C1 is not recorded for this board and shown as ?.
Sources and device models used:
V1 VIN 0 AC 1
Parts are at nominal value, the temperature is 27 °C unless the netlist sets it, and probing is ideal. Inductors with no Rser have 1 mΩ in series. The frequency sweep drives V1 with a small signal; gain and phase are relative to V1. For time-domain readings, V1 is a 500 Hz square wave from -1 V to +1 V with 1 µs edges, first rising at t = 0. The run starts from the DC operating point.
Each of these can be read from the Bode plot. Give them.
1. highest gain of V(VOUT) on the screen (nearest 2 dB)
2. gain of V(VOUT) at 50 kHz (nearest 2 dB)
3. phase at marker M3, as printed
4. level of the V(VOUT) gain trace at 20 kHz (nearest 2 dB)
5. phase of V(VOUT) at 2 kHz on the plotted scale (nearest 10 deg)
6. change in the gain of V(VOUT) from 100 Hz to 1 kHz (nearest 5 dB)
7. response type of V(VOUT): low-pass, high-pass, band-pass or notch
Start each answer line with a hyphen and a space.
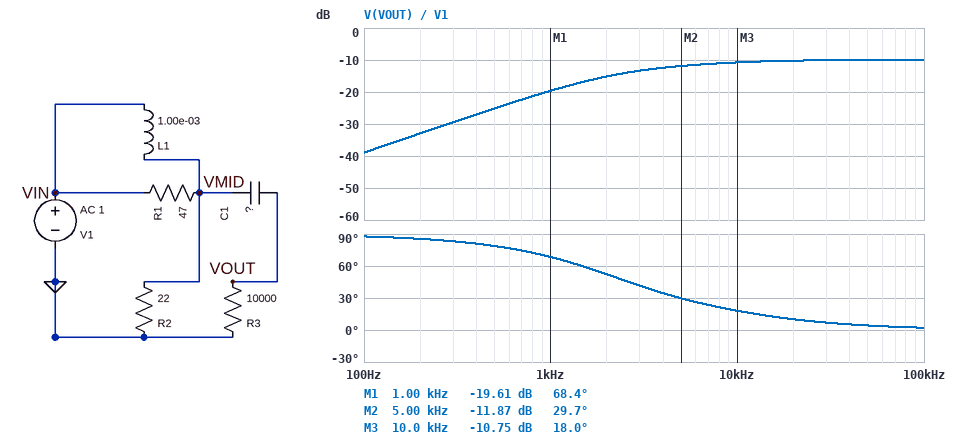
- -10 dB
- -10 dB
- 18.0 deg
- -10 dB
- 50 deg
- 20 dB
- high-pass
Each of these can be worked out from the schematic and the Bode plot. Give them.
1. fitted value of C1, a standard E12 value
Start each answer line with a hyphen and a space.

- 1.8 nF
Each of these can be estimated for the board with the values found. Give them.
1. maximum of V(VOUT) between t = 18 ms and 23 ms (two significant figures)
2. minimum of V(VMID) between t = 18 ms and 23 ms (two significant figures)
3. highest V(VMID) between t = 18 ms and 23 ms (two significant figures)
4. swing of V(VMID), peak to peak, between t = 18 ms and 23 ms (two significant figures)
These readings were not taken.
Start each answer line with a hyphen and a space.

- 630 mV
- -1.0 V
- 1.0 V
- 2.0 V
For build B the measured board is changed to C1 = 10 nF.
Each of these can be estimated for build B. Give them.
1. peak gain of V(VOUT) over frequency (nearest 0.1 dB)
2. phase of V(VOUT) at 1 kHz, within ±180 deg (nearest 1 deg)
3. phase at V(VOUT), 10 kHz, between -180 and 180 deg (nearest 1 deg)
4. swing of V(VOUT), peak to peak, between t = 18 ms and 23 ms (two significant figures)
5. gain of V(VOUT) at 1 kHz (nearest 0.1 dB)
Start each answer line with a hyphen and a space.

- -4.1 dB
- 43 deg
- -14 deg
- 1.9 V
- -6.1 dB
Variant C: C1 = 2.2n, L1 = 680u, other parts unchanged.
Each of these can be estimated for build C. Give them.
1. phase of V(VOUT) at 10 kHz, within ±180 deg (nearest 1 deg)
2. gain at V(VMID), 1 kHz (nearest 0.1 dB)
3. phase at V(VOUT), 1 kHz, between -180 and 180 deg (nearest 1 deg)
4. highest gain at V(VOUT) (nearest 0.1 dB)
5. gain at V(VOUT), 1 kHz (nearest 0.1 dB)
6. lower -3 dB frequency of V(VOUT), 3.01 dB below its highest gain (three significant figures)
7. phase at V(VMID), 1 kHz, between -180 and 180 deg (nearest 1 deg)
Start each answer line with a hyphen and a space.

- 7 deg
- -0.3 dB
- 71 deg
- -8.7 dB
- -17.6 dB
- 2.33 kHz
- -11 deg
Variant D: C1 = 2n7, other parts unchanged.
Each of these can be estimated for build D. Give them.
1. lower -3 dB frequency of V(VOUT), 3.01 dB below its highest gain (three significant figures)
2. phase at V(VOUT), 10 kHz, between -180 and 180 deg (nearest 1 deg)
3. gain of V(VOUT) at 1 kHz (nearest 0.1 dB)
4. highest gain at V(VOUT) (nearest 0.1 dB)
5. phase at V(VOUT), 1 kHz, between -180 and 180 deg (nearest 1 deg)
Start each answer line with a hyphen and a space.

- 1.79 kHz
- 7 deg
- -16.2 dB
- -9.4 dB
- 65 deg
